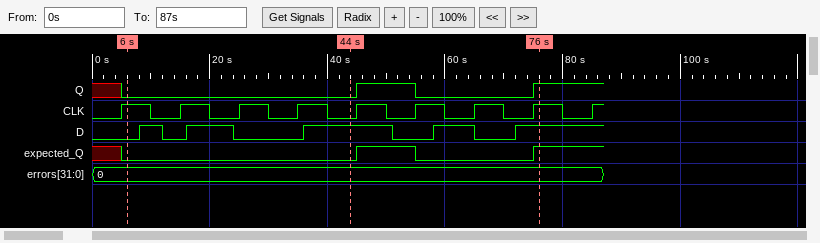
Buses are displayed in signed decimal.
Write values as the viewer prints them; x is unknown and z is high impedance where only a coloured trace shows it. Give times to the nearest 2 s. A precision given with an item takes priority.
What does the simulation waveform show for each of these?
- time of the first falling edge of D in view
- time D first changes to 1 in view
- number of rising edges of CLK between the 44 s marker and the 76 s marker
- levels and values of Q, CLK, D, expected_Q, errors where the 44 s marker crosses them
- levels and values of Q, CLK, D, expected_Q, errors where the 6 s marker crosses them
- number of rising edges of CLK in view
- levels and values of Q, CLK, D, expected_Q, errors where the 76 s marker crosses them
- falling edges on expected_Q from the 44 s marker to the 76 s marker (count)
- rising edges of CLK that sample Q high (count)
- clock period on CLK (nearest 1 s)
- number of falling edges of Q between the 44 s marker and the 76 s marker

12 s
8 s
4
Q=0, CLK=0, D=1, expected_Q=0, errors=0
Q=0, CLK=1, D=0, expected_Q=0, errors=0
9
Q=1, CLK=1, D=1, expected_Q=1, errors=0
1
2
10 s
1
